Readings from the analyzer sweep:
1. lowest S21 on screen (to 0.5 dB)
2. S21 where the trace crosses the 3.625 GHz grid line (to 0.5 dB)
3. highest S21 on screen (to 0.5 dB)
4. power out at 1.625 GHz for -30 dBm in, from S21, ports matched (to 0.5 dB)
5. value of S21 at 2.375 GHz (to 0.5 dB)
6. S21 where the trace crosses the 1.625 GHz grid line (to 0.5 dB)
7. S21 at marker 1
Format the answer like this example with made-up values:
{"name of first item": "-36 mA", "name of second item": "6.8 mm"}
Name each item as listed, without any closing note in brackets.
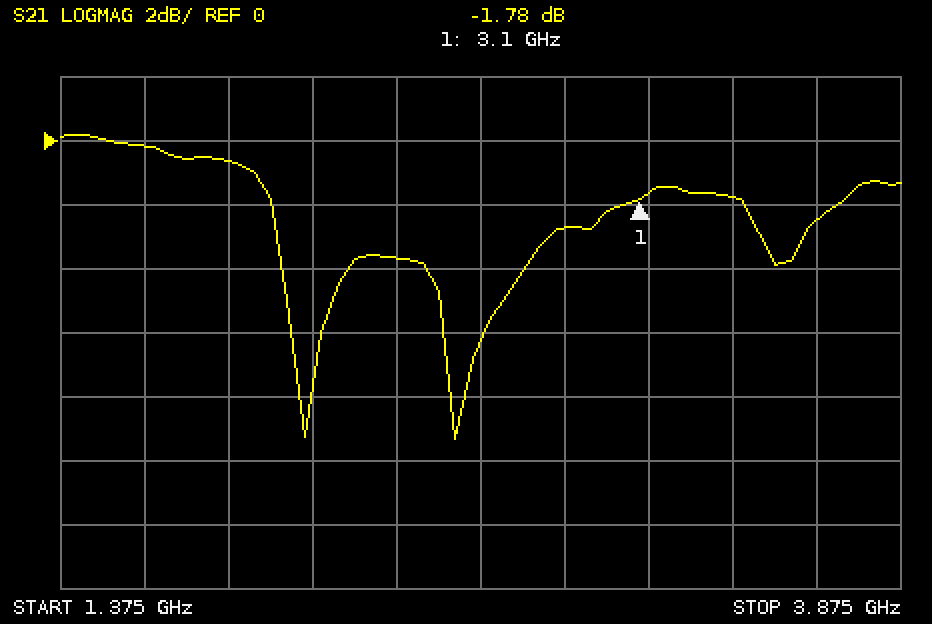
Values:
{"lowest S21 on screen": "-9.5 dB", "S21 where the trace crosses the 3.625 GHz grid line": "-2.5 dB", "highest S21 on screen": "0.0 dB", "power out at 1.625 GHz for -30 dBm in, from S21, ports matched": "-30.0 dBm", "value of S21 at 2.375 GHz": "-3.5 dB", "S21 where the trace crosses the 1.625 GHz grid line": "0.0 dB", "S21 at marker 1": "-1.78 dB"}
